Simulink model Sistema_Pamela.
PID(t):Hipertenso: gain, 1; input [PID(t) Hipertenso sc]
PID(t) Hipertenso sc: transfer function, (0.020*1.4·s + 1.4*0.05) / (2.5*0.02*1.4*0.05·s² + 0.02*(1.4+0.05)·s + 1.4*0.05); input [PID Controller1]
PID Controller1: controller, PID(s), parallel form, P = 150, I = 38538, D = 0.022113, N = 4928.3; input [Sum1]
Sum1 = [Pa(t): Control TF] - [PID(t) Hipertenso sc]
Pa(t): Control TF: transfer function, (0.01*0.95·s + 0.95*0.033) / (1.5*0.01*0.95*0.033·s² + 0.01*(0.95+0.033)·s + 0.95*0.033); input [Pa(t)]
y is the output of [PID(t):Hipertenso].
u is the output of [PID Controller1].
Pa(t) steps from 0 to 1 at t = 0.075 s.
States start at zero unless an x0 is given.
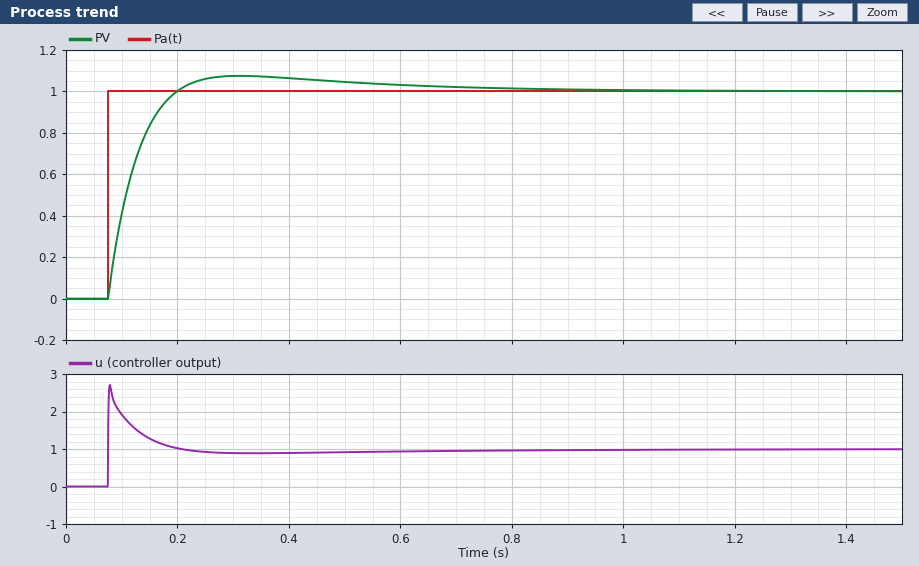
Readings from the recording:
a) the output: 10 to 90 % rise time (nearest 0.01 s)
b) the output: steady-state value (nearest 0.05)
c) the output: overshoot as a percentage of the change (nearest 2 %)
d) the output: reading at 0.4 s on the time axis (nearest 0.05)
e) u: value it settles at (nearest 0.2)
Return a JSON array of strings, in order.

["0.08 s", "1.00", "8 %", "1.05", "1.0"]
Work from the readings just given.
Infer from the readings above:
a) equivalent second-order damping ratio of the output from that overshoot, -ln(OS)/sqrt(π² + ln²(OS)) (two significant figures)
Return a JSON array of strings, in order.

["0.63"]
